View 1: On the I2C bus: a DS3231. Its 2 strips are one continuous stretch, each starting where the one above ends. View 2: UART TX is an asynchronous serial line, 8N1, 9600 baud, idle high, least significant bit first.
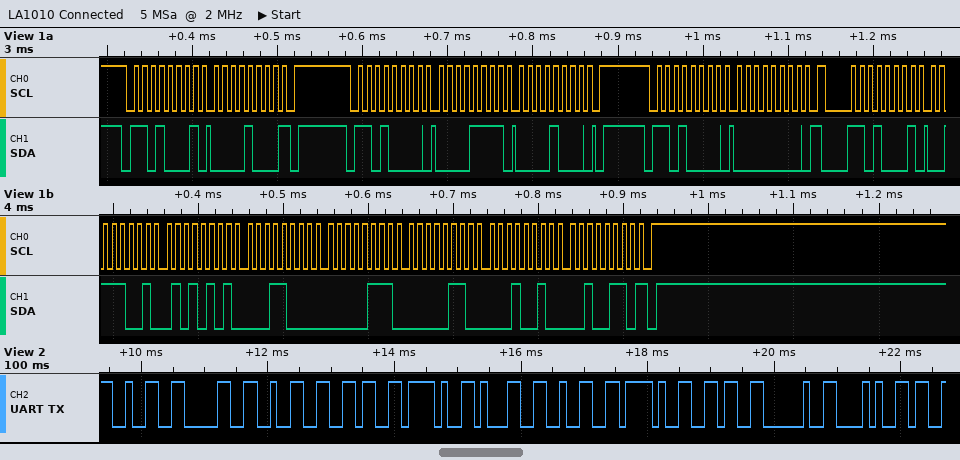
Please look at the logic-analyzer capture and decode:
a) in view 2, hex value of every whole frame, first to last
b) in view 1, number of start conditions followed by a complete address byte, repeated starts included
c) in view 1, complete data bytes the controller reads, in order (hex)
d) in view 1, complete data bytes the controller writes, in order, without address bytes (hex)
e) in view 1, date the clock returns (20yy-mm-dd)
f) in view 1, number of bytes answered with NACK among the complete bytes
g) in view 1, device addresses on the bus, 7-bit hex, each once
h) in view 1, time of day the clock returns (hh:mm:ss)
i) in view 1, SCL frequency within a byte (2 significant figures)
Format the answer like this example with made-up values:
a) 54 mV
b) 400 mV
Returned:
a) 0x32 0x30 0x32 0x36 0x2F 0x31 0x32 0x2F 0x36 0x20 0x28
b) 4
c) 08 39 55 18 07 06 12 26
d) 0F 08 00
e) 2026-12-06
f) 2
g) 0x68
h) 18:55:39
i) 100 kHz
